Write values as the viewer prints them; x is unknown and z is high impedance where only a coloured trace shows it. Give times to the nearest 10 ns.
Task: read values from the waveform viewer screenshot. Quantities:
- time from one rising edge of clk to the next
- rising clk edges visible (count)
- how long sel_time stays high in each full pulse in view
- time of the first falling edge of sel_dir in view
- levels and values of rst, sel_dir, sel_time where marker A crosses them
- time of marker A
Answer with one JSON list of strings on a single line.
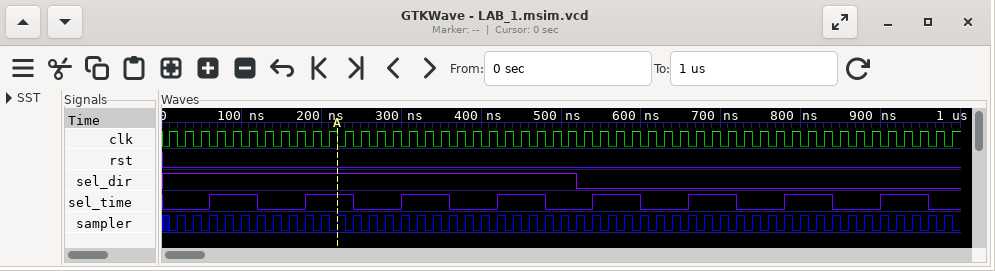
["20 ns", "50", "60 ns, 60 ns, 60 ns, 60 ns, 60 ns, 60 ns, 60 ns, 60 ns", "520 ns", "rst=0, sel_dir=1, sel_time=1", "220 ns"]
